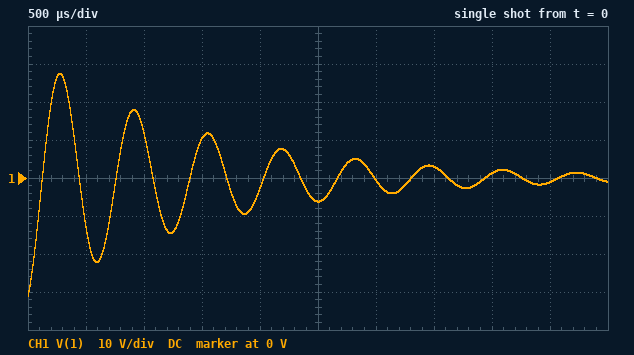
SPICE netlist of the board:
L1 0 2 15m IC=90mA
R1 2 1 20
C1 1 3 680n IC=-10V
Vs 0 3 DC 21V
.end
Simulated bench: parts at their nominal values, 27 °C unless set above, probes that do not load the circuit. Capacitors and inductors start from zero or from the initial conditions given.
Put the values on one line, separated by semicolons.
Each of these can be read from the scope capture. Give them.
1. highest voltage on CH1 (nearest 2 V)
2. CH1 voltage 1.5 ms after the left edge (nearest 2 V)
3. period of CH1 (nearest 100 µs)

28 V; 10 V; 600 µs
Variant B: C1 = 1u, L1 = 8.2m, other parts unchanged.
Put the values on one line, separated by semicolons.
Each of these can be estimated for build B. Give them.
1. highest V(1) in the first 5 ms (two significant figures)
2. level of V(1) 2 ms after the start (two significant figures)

23 V; 2.7 V
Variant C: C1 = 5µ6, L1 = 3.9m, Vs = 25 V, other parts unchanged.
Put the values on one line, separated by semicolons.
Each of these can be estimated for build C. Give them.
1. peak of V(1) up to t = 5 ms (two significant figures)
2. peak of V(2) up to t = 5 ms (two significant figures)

9.7 V; 13 V
